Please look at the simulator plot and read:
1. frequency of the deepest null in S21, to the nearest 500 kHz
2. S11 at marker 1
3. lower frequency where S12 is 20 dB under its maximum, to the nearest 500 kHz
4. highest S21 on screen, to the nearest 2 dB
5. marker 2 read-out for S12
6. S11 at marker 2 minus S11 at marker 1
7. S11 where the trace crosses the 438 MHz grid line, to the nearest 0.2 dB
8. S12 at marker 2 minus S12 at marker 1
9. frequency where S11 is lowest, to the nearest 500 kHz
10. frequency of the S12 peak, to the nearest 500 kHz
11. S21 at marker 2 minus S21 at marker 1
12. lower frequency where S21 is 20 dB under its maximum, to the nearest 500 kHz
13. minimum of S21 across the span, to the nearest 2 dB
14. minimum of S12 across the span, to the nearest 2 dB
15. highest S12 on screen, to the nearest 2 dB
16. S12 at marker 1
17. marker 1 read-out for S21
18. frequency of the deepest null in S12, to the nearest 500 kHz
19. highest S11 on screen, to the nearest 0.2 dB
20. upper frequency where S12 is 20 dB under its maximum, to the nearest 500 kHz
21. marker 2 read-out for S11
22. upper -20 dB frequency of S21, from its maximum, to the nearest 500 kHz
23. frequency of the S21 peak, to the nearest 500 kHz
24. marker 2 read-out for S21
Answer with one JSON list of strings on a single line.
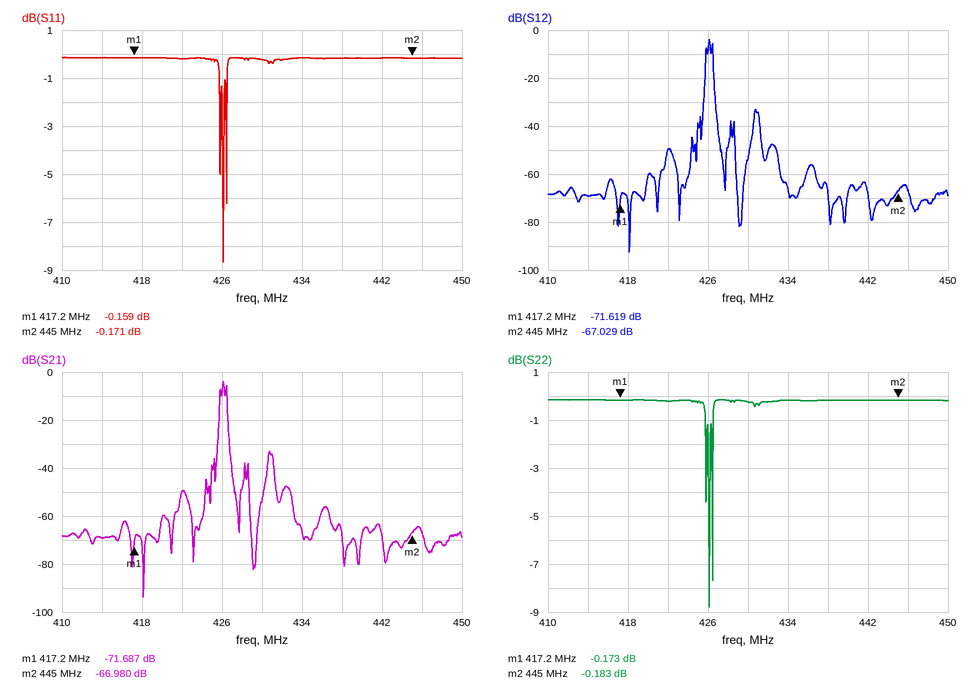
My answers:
["418.0 MHz", "-0.159 dB", "425.5 MHz", "-4 dB", "-67.029 dB", "-0.012 dB", "-0.2 dB", "4.590 dB", "426.0 MHz", "426.0 MHz", "4.707 dB", "425.5 MHz", "-94 dB", "-92 dB", "-4 dB", "-71.619 dB", "-71.687 dB", "418.0 MHz", "-0.2 dB", "426.5 MHz", "-0.171 dB", "426.5 MHz", "426.0 MHz", "-66.980 dB"]
